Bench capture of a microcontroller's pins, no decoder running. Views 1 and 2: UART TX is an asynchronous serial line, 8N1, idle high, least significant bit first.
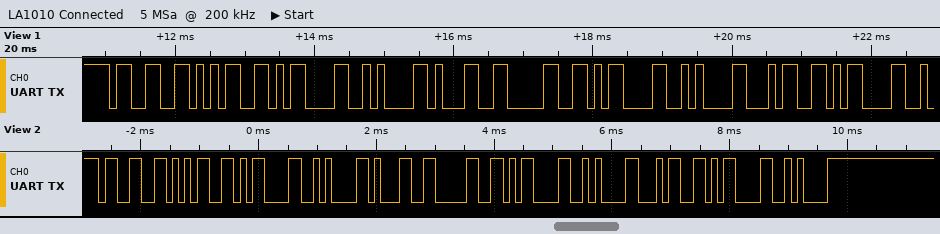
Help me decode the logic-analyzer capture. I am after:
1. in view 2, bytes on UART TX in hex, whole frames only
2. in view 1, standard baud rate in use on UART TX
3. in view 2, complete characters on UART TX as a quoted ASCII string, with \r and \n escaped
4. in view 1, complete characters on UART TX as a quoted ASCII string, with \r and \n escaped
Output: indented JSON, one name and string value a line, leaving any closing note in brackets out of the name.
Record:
{
  "in view 2, bytes on UART TX in hex, whole frames only": "33 35 0D 0A 31 30 0D 0A 34 0D 0A",
  "in view 1, standard baud rate in use on UART TX": "9600 baud",
  "in view 2, complete characters on UART TX as a quoted ASCII string, with \\r and \\n escaped": "\"35\\r\\n10\\r\\n4\\r\\n\"",
  "in view 1, complete characters on UART TX as a quoted ASCII string, with \\r and \\n escaped": "\"35\\r\\n10\\r\\n4\\r\""
}
